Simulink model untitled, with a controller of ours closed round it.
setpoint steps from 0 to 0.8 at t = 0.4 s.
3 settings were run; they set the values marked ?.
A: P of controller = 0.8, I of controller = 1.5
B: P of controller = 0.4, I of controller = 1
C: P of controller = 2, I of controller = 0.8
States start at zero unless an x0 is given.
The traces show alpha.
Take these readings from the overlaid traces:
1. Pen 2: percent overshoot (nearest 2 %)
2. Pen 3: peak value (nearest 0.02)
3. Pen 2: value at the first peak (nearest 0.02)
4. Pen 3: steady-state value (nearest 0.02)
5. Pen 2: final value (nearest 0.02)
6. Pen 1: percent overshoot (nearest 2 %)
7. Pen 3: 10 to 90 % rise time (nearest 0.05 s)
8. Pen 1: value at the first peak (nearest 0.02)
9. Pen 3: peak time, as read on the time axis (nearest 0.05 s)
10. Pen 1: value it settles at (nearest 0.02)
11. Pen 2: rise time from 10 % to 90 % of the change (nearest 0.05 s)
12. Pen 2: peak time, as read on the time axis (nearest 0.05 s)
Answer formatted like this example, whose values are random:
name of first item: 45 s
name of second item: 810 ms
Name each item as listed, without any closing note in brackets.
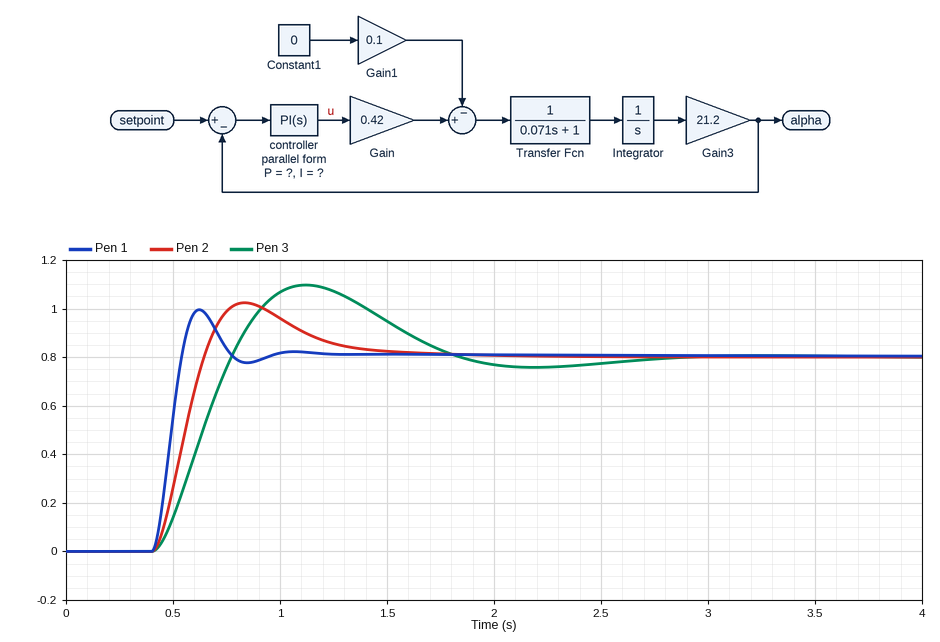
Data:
Pen 2: percent overshoot: 28 %
Pen 3: peak value: 1.10
Pen 2: value at the first peak: 1.02
Pen 3: steady-state value: 0.80
Pen 2: final value: 0.80
Pen 1: percent overshoot: 24 %
Pen 3: 10 to 90 % rise time: 0.25 s
Pen 1: value at the first peak: 1.00
Pen 3: peak time, as read on the time axis: 1.10 s
Pen 1: value it settles at: 0.80
Pen 2: rise time from 10 % to 90 % of the change: 0.15 s
Pen 2: peak time, as read on the time axis: 0.85 s
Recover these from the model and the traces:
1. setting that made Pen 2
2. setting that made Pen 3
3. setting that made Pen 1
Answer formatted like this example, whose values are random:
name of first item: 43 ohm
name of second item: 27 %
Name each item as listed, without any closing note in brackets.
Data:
setting that made Pen 2: A
setting that made Pen 3: B
setting that made Pen 1: C
